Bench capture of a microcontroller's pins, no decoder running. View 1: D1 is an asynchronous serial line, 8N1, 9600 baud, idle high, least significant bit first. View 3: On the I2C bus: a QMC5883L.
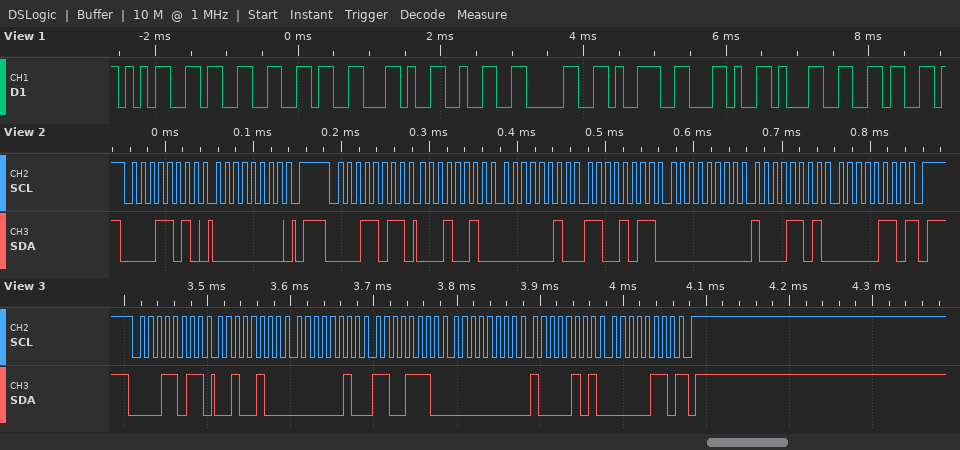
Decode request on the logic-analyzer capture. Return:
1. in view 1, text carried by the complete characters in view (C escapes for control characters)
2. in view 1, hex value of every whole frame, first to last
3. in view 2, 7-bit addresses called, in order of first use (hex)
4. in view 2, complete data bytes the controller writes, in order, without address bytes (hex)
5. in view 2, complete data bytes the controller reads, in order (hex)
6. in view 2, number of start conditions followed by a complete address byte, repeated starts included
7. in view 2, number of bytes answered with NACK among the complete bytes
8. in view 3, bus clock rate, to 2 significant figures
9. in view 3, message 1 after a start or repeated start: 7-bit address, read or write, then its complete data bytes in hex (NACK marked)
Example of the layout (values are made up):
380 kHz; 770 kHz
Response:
"536,209,16"; 35 33 36 2C 32 30 39 2C 31 36; 0x0D; 00; 12 02 CB 00 8D 06; 2; 1; 100 kHz; 0x0D read: 24 02 CE 00 85 06 NACK
